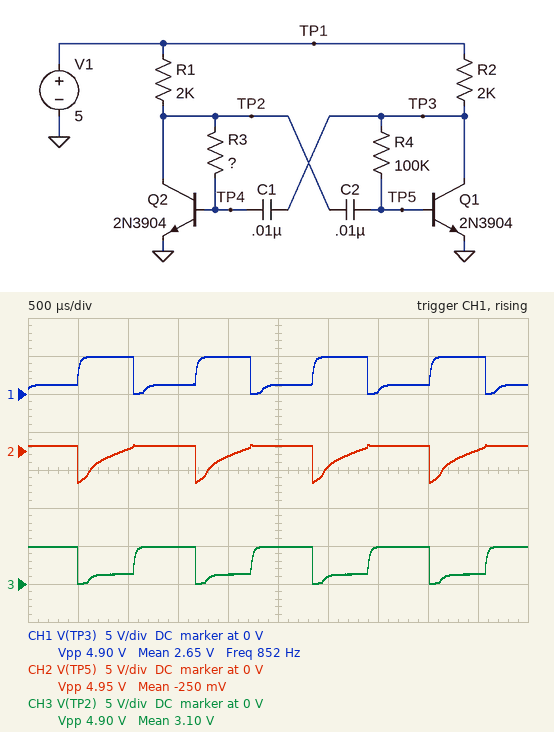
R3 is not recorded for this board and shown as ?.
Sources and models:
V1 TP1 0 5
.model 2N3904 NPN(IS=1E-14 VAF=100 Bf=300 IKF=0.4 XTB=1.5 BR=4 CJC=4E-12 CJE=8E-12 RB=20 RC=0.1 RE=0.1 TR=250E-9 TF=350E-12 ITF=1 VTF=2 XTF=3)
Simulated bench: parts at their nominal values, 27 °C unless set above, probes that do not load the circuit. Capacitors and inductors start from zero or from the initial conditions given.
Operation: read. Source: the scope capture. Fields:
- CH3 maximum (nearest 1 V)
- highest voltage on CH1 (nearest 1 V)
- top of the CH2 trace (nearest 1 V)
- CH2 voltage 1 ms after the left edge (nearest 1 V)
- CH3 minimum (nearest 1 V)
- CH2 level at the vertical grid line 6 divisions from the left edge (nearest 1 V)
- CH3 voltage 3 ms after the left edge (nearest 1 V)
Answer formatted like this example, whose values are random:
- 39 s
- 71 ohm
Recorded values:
- 5 V
- 5 V
- 1 V
- 0 V
- 0 V
- -2 V
- 1 V
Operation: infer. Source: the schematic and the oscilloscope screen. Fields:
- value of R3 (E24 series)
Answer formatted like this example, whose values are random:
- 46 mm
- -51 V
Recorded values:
- 110 kΩ
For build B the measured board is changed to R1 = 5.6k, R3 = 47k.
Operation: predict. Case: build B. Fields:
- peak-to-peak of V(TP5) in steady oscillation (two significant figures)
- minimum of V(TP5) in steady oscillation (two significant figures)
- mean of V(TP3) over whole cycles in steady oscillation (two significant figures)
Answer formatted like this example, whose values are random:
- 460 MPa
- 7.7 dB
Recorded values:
- 4.5 V
- -3.8 V
- 2.9 V
